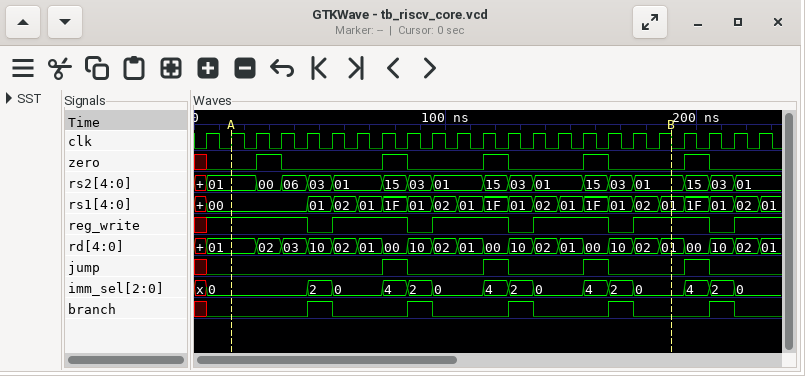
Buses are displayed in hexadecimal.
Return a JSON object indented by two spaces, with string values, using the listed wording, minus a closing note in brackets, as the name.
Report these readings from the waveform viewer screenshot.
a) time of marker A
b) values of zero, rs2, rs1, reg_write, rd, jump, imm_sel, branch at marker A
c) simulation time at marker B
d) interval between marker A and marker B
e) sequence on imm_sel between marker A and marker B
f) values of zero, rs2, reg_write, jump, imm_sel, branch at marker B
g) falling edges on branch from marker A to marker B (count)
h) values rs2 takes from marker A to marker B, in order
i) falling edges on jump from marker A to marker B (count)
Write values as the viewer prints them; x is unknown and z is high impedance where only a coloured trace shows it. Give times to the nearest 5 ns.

{
  "time of marker A": "15 ns",
  "values of zero, rs2, rs1, reg_write, rd, jump, imm_sel, branch at marker A": "zero=0, rs2=01, rs1=00, reg_write=1, rd=01, jump=0, imm_sel=0, branch=0",
  "simulation time at marker B": "190 ns",
  "interval between marker A and marker B": "175 ns",
  "sequence on imm_sel between marker A and marker B": "0, 2, 0, 4, 2, 0, 4, 2, 0, 4, 2, 0",
  "values of zero, rs2, reg_write, jump, imm_sel, branch at marker B": "zero=0, rs2=01, reg_write=1, jump=0, imm_sel=0, branch=0",
  "falling edges on branch from marker A to marker B": "4",
  "values rs2 takes from marker A to marker B, in order": "01, 00, 06, 03, 01, 15, 03, 01, 15, 03, 01, 15, 03, 01",
  "falling edges on jump from marker A to marker B": "3"
}
